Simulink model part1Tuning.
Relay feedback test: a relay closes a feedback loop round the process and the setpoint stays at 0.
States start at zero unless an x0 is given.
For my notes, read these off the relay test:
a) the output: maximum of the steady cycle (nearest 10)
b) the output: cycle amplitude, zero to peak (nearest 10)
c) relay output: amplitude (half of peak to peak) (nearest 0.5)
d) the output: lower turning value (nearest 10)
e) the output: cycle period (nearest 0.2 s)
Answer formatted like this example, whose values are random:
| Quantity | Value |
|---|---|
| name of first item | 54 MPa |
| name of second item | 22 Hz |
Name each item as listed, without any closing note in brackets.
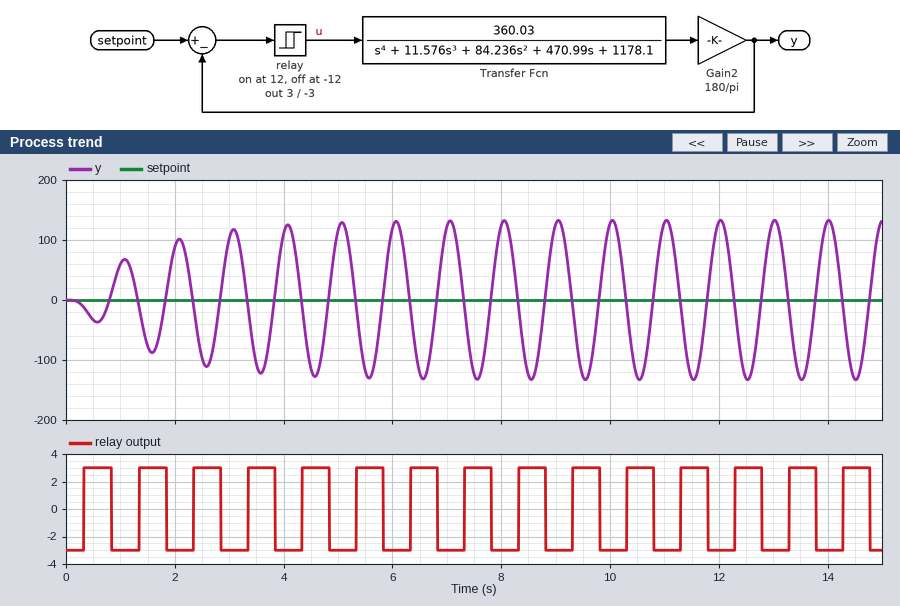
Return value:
| Quantity | Value |
|---|---|
| the output: maximum of the steady cycle | 130 |
| the output: cycle amplitude, zero to peak | 130 |
| relay output: amplitude (half of peak to peak) | 3.0 |
| the output: lower turning value | -130 |
| the output: cycle period | 1.0 s |
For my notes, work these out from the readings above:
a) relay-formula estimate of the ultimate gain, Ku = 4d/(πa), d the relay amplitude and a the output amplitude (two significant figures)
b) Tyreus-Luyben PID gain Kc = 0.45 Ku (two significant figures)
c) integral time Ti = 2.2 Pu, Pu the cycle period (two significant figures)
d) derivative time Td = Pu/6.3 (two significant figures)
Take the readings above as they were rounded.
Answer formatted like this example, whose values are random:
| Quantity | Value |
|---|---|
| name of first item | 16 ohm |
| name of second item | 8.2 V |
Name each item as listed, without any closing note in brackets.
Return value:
| Quantity | Value |
|---|---|
| relay-formula estimate of the ultimate gain, Ku = 4d/(πa), d the relay amplitude and a the output amplitude | 0.029 |
| Tyreus-Luyben PID gain Kc = 0.45 Ku | 0.013 |
| integral time Ti = 2.2 Pu, Pu the cycle period | 2.2 s |
| derivative time Td = Pu/6.3 | 0.16 s |
